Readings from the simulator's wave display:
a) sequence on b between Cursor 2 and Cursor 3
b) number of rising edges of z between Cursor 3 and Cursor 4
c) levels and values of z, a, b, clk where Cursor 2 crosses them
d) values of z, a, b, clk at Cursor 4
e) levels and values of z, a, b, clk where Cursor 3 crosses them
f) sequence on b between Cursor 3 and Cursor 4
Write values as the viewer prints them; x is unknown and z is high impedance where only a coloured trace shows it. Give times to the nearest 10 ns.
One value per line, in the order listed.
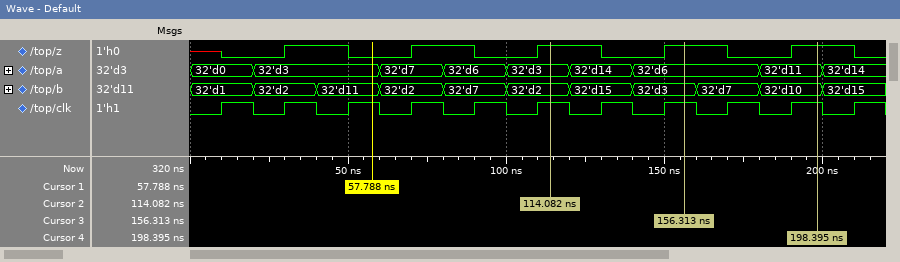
32'd2, 32'd15, 32'd3
1
z=1, a=32'd3, b=32'd2, clk=1
z=1, a=32'd11, b=32'd10, clk=1
z=1, a=32'd6, b=32'd3, clk=1
32'd3, 32'd7, 32'd10
